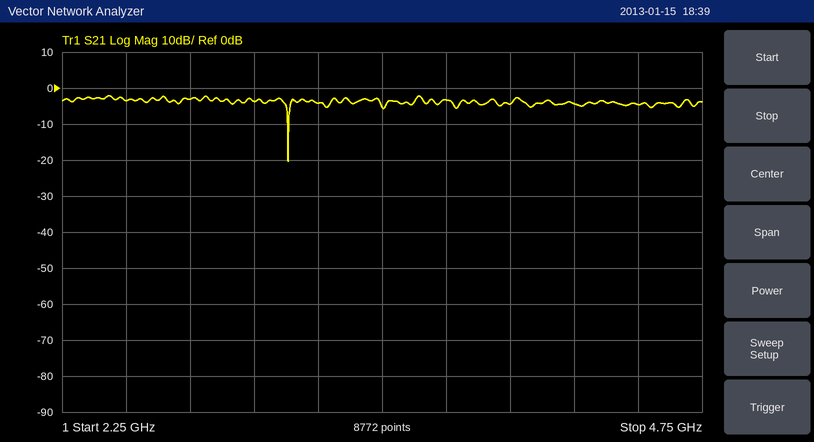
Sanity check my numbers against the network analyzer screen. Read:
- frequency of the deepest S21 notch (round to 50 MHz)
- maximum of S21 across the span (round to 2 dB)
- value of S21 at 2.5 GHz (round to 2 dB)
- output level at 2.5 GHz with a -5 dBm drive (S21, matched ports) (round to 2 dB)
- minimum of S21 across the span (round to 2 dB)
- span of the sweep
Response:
3.15 GHz
-2 dB
-4 dB
-8 dBm
-20 dB
2.5 GHz
